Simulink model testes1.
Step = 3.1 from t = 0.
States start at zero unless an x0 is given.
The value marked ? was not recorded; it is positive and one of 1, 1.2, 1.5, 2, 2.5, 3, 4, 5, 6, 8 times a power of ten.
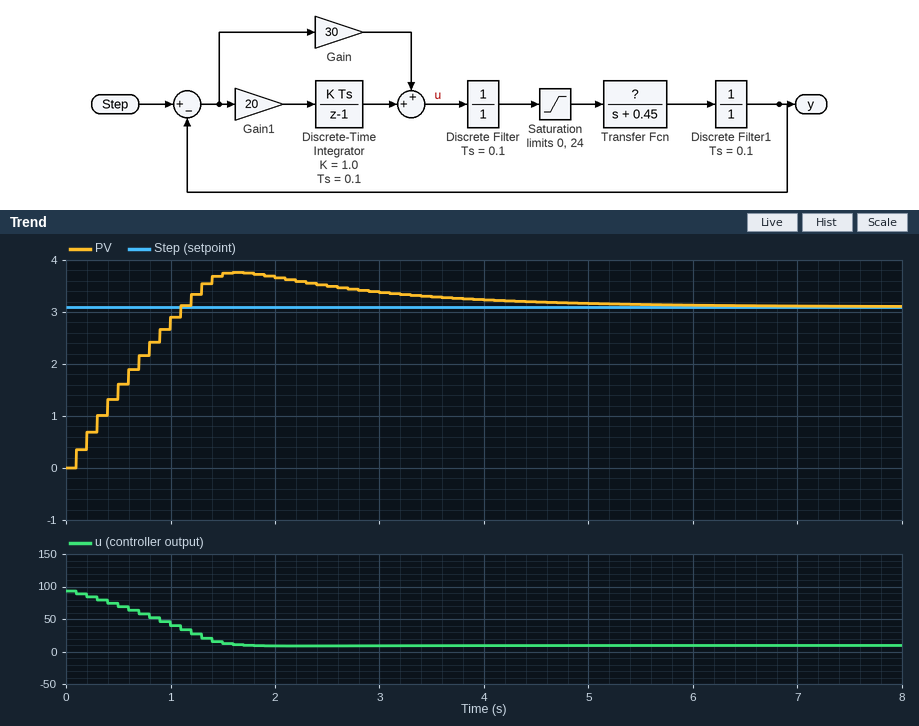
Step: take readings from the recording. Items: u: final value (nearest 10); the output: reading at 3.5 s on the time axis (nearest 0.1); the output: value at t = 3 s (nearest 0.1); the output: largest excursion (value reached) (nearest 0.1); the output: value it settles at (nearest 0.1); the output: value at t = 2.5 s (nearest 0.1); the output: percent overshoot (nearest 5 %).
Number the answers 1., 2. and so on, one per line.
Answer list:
1. 10
2. 3.3
3. 3.4
4. 3.8
5. 3.1
6. 3.5
7. 20 %
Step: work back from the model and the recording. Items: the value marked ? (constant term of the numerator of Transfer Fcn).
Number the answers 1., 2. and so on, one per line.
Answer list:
1. 0.15
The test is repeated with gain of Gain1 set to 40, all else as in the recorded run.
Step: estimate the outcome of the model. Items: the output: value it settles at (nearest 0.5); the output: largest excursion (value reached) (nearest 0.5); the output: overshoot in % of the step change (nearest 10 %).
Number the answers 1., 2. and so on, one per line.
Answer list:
1. 3.0
2. 4.5
3. 40 %
